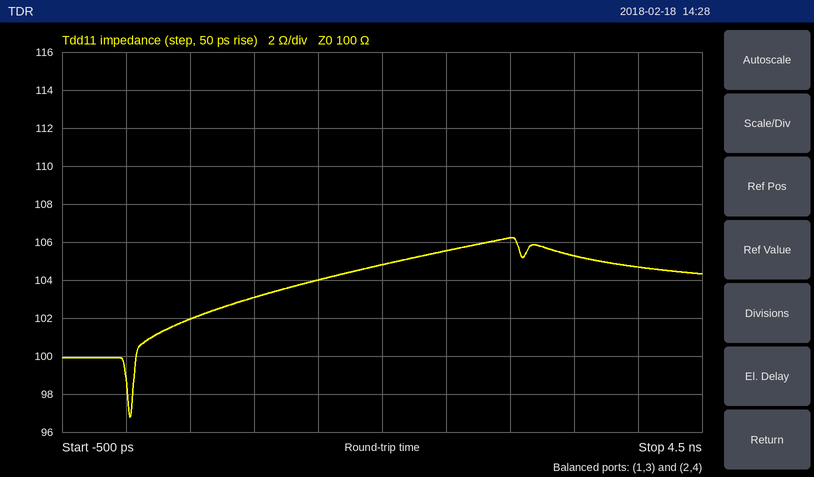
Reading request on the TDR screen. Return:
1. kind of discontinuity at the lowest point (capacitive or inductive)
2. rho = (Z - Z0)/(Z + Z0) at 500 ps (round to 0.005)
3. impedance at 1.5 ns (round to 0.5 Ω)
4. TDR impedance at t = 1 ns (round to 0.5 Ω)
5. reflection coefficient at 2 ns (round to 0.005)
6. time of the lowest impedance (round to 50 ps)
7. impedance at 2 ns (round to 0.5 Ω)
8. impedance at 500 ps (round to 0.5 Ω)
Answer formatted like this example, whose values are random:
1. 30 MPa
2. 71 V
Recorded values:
1. capacitive
2. +0.010
3. 104.0 Ω
4. 103.0 Ω
5. +0.025
6. 50 ps
7. 105.0 Ω
8. 102.0 Ω
